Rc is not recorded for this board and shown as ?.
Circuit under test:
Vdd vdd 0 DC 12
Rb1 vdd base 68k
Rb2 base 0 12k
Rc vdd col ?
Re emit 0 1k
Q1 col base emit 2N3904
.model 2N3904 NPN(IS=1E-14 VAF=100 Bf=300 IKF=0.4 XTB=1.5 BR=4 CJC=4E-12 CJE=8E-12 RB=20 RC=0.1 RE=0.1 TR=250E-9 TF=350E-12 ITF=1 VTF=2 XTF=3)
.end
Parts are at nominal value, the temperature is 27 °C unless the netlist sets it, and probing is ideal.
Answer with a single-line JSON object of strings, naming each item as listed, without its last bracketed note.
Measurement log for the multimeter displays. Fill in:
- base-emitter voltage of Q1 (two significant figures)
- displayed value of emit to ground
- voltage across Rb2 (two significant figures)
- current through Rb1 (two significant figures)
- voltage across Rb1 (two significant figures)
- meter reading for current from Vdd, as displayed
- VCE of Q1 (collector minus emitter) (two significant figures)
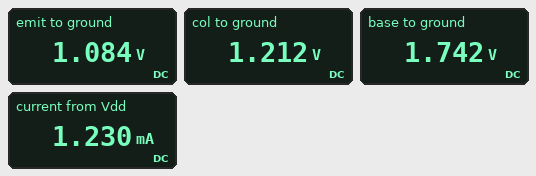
{"base-emitter voltage of Q1": "660 mV", "displayed value of emit to ground": "1.084 V", "voltage across Rb2": "1.7 V", "current through Rb1": "150 µA", "voltage across Rb1": "10 V", "meter reading for current from Vdd, as displayed": "1.230 mA", "VCE of Q1 (collector minus emitter)": "130 mV"}
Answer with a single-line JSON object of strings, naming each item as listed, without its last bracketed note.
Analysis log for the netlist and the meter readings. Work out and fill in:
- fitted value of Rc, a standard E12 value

{"fitted value of Rc, a standard E12 value": "10 kΩ"}
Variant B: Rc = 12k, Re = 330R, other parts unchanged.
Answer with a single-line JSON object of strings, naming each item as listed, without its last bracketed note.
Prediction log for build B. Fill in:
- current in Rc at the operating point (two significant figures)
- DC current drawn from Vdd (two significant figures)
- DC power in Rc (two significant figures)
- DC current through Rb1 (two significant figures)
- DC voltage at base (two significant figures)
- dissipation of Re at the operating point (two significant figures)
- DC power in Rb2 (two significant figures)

{"current in Rc at the operating point": "970 µA", "DC current drawn from Vdd": "1.1 mA", "DC power in Rc": "11 mW", "DC current through Rb1": "160 µA", "DC voltage at base": "1.0 V", "dissipation of Re at the operating point": "360 µW", "DC power in Rb2": "85 µW"}
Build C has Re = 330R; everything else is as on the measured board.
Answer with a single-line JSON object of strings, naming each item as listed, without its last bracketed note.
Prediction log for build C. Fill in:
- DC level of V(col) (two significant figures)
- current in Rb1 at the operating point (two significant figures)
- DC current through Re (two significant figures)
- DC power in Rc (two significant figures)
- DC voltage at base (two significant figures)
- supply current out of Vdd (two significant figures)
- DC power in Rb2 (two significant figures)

{"DC level of V(col)": "450 mV", "current in Rb1 at the operating point": "160 µA", "DC current through Re": "1.2 mA", "DC power in Rc": "13 mW", "DC voltage at base": "1.1 V", "supply current out of Vdd": "1.3 mA", "DC power in Rb2": "96 µW"}
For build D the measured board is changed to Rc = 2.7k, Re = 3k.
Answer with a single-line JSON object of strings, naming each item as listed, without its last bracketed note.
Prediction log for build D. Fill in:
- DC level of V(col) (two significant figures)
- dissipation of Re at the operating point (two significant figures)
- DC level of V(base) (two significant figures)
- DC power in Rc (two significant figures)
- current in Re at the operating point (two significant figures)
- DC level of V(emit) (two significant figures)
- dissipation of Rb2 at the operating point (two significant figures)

{"DC level of V(col)": "11 V", "dissipation of Re at the operating point": "450 µW", "DC level of V(base)": "1.8 V", "DC power in Rc": "400 µW", "current in Re at the operating point": "390 µA", "DC level of V(emit)": "1.2 V", "dissipation of Rb2 at the operating point": "270 µW"}
